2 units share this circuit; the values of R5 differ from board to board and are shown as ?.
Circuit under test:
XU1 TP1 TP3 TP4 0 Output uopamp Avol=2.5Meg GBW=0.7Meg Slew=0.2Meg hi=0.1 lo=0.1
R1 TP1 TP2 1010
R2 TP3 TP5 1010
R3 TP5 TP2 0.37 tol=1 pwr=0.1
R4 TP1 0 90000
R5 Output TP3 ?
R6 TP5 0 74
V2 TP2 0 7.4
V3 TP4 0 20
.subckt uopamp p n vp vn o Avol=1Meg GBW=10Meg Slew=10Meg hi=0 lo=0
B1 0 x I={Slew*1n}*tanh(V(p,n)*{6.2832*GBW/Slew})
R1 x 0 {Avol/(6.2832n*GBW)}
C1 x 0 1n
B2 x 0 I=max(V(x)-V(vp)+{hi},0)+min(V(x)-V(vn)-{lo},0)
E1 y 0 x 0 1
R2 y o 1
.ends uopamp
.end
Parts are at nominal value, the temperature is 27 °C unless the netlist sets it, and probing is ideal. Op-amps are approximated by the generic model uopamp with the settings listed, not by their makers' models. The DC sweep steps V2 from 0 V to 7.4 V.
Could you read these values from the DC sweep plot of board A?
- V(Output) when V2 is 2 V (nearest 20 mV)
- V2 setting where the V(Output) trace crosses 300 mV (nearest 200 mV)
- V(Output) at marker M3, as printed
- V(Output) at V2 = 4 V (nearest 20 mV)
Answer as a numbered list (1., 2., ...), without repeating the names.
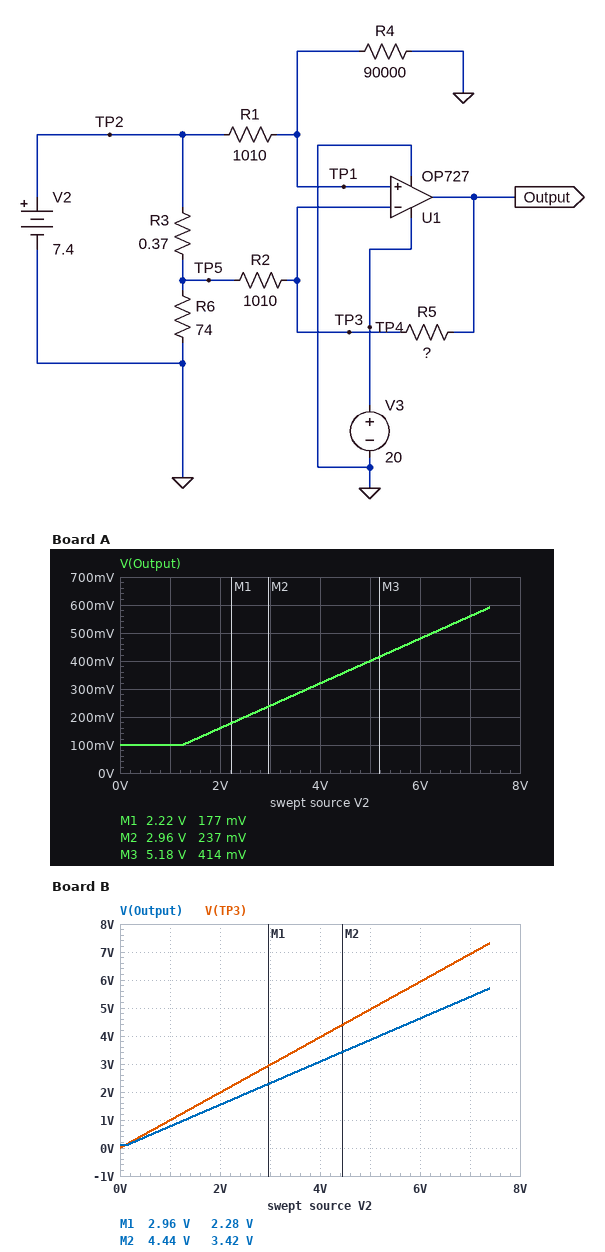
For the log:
1. 160 mV
2. 3.8 V
3. 414 mV
4. 320 mV
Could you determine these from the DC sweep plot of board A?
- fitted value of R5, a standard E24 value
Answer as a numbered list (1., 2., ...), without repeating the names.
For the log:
1. 150 kΩ
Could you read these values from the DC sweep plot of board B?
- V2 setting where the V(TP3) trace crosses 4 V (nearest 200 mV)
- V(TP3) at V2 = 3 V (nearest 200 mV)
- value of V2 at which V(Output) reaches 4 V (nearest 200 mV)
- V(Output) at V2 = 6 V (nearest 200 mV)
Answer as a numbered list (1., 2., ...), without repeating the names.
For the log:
1. 4.0 V
2. 3.0 V
3. 5.2 V
4. 4.6 V
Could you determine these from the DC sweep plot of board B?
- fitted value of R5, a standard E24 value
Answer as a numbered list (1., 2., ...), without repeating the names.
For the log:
1. 36 kΩ
